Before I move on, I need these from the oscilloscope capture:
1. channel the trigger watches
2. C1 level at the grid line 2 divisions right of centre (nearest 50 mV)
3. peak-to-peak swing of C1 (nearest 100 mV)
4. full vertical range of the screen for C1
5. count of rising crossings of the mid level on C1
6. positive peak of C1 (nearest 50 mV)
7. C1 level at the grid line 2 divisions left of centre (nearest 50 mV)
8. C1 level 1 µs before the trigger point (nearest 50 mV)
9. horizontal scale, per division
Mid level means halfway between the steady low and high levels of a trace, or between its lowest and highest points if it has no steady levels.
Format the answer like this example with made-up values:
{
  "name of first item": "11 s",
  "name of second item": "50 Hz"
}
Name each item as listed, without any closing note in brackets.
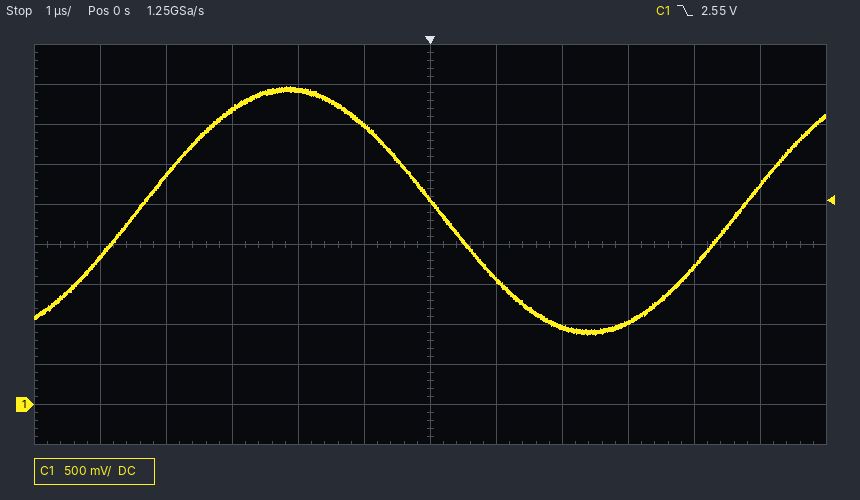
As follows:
{
  "channel the trigger watches": "C1",
  "C1 level at the grid line 2 divisions right of centre": "950 mV",
  "peak-to-peak swing of C1": "3.10 V",
  "full vertical range of the screen for C1": "5 V",
  "count of rising crossings of the mid level on C1": "2",
  "positive peak of C1": "4.00 V",
  "C1 level at the grid line 2 divisions left of centre": "3.95 V",
  "C1 level 1 µs before the trigger point": "3.50 V",
  "horizontal scale, per division": "1 µs"
}
